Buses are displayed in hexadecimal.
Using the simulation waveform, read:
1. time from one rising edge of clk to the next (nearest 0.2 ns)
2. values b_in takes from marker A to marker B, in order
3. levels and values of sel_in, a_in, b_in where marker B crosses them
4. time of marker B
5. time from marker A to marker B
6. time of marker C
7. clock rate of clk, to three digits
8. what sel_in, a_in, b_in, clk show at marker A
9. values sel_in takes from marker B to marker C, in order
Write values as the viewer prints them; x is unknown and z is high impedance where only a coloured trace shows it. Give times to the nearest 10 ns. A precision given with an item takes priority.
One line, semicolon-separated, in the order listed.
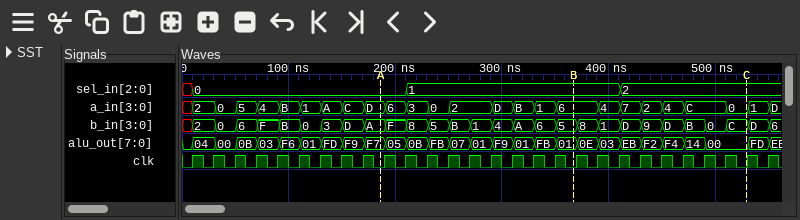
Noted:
20 ns; A, F, 8, 5, B, 1, 4, A, 6, 5; sel_in=1, a_in=6, b_in=5; 370 ns; 180 ns; 530 ns; 50.0 MHz; sel_in=0, a_in=D, b_in=A, clk=0; 1, 2
